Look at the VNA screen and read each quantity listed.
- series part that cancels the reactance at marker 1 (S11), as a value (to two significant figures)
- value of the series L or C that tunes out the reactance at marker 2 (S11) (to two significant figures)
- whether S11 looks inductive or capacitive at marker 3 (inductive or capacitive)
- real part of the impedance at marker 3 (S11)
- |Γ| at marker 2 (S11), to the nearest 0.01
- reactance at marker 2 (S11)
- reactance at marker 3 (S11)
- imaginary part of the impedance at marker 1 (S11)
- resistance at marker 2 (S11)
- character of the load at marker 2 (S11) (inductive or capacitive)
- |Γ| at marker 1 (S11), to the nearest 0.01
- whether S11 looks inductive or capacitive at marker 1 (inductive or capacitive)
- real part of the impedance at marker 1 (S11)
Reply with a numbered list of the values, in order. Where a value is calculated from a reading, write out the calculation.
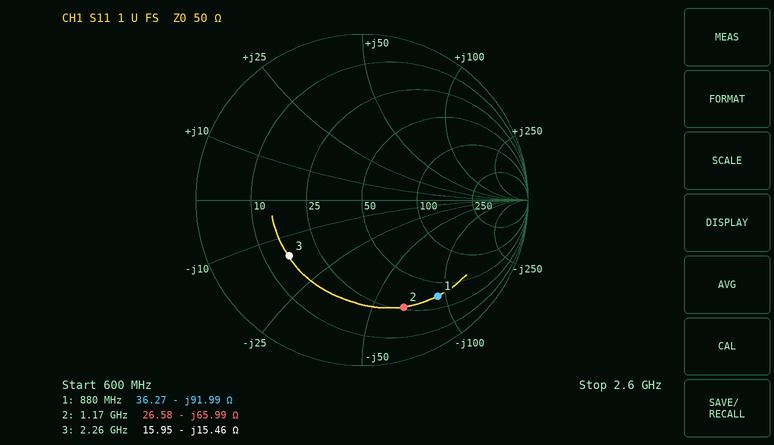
1. L = 91.99 Ω/(2π × 880 MHz) ≈ 17 nH
2. L = 65.99 Ω/(2π × 1.17 GHz) ≈ 9.0 nH
3. capacitive
4. 15.95 Ω
5. 0.69
6. -65.99 Ω
7. -15.46 Ω
8. -91.99 Ω
9. 26.58 Ω
10. capacitive
11. 0.74
12. capacitive
13. 36.27 Ω
